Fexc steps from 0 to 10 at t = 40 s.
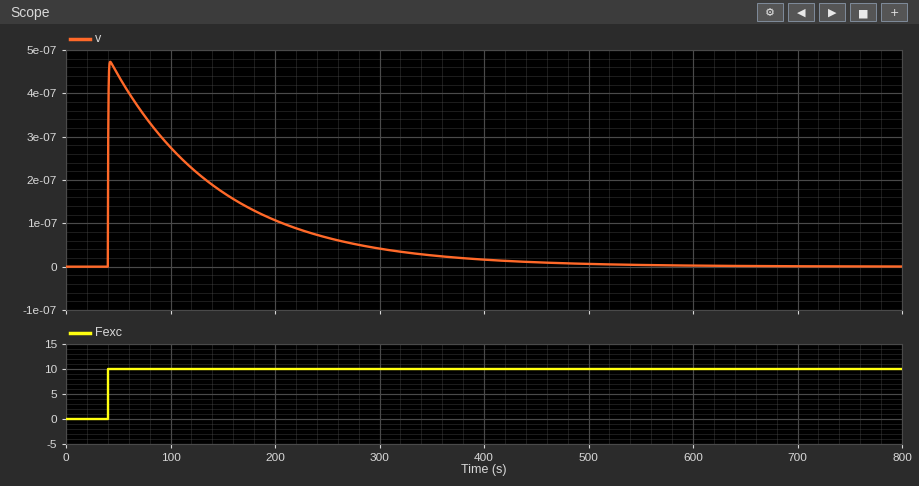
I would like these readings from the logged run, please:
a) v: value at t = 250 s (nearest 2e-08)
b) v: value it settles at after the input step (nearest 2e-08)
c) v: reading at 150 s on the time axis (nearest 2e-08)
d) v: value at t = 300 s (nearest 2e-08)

0.00000006
0.00000000
0.00000018
0.00000004
